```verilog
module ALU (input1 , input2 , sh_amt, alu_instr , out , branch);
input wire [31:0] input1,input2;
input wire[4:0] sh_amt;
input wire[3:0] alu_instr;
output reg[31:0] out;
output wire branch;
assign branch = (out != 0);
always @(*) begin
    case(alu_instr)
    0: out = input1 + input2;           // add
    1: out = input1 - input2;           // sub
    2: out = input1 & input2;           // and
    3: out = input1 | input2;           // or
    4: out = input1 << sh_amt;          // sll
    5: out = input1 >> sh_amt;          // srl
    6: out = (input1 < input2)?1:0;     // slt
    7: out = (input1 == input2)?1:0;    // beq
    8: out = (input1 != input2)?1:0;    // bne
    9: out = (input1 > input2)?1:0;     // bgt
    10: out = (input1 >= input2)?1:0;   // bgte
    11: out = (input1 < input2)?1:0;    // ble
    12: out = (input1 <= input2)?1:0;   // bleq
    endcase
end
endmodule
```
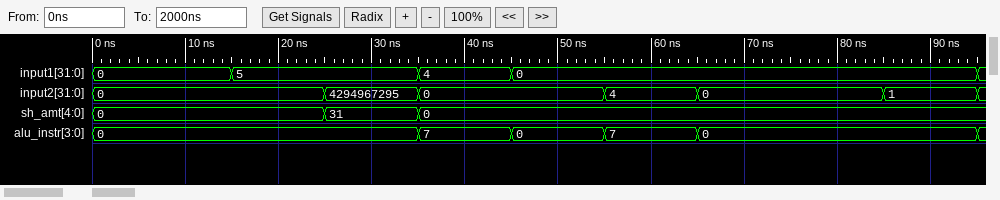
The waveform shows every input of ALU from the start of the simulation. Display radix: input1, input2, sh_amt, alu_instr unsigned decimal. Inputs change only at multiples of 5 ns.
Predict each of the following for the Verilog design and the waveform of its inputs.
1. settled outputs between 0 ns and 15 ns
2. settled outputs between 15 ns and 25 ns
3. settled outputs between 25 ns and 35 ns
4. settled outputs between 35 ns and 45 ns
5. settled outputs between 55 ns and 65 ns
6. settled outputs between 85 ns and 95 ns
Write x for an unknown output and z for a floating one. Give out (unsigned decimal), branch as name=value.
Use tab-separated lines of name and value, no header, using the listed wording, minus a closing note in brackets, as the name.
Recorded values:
settled outputs between 0 ns and 15 ns	out=0, branch=0
settled outputs between 15 ns and 25 ns	out=5, branch=1
settled outputs between 25 ns and 35 ns	out=4, branch=1
settled outputs between 35 ns and 45 ns	out=0, branch=0
settled outputs between 55 ns and 65 ns	out=0, branch=0
settled outputs between 85 ns and 95 ns	out=1, branch=1
